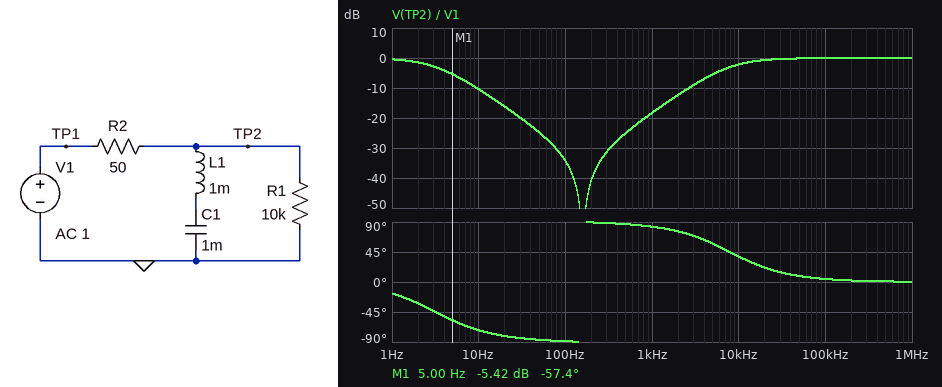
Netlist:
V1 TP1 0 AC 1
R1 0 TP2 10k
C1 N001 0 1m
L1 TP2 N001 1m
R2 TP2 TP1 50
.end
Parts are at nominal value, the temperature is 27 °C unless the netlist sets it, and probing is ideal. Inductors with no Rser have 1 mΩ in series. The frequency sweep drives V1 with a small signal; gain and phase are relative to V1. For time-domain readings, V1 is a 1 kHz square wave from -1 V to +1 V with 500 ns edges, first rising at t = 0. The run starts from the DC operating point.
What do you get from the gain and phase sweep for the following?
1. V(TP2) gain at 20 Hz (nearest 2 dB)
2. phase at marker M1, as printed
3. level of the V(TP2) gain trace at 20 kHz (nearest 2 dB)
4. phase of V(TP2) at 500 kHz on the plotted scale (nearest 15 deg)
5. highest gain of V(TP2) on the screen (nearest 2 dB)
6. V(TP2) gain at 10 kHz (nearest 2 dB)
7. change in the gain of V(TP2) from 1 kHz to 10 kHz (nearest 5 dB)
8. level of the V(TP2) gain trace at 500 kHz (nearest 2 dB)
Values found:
-16 dB
-57.4 deg
0 dB
0 deg
0 dB
-2 dB
15 dB
0 dB
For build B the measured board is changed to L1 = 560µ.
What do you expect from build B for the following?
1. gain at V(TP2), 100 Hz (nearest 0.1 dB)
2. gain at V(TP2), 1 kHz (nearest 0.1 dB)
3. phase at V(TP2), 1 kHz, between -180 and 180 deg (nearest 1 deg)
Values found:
-32.1 dB
-23.5 dB
86 deg
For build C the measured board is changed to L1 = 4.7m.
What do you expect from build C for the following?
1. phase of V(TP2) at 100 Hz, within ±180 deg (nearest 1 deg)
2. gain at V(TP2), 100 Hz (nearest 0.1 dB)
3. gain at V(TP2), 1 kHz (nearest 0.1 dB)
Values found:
88 deg
-31.3 dB
-5.9 dB
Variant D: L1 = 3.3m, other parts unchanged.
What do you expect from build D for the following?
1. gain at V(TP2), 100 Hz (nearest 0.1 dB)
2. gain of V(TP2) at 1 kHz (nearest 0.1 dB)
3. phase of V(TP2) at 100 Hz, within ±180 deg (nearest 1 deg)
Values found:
-40.3 dB
-8.4 dB
89 deg
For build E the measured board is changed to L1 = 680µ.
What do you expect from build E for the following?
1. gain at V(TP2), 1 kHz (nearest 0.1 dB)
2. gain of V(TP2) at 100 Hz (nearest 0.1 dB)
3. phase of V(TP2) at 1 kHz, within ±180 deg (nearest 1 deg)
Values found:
-21.7 dB
-32.7 dB
85 deg
